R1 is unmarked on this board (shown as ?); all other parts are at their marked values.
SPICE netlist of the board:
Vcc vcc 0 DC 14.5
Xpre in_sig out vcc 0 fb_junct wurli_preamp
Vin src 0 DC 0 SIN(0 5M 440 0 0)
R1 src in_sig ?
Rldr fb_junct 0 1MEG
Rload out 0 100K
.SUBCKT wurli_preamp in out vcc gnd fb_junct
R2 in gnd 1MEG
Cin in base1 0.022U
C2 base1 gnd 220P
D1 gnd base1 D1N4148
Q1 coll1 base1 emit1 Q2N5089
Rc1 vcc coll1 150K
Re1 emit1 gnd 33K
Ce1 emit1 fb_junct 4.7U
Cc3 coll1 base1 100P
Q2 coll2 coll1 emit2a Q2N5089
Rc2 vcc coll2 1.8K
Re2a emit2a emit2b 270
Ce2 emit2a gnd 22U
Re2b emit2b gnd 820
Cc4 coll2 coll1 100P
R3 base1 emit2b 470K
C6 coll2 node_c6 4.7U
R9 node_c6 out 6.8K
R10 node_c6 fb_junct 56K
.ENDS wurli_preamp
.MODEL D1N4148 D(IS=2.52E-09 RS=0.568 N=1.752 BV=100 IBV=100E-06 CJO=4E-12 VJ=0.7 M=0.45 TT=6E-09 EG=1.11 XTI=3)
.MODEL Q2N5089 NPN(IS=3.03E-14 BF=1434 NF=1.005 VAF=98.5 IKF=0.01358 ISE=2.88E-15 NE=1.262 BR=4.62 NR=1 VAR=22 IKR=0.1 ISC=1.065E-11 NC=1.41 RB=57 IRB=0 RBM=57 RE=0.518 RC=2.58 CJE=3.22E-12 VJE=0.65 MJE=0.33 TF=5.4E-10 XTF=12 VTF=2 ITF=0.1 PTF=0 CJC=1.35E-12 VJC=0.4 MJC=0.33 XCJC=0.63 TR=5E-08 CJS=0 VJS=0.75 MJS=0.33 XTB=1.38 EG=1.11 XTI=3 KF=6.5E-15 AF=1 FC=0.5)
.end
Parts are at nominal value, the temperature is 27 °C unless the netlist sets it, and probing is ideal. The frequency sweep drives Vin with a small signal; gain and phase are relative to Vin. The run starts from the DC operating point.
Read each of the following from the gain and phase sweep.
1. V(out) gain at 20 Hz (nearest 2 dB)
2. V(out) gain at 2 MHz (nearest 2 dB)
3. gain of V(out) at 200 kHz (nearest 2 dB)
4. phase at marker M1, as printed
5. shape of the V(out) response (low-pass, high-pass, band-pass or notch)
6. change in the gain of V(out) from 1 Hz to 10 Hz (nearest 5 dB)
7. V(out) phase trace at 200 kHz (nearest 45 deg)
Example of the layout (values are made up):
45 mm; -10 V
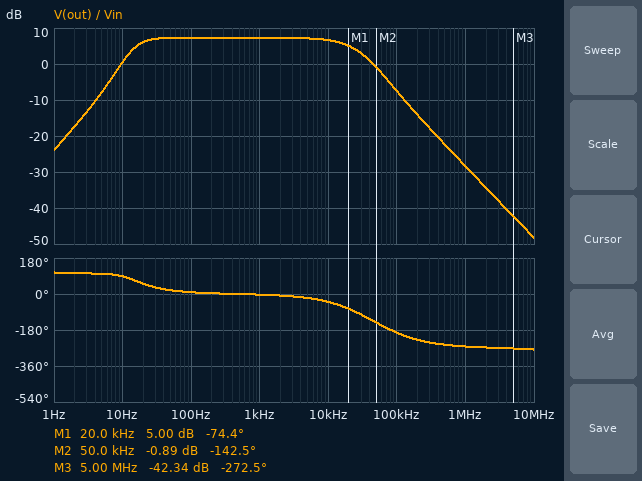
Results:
6 dB; -34 dB; -14 dB; -74.4 deg; band-pass; 25 dB; -225 deg
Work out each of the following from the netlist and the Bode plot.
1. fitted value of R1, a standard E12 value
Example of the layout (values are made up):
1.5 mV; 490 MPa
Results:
12 kΩ
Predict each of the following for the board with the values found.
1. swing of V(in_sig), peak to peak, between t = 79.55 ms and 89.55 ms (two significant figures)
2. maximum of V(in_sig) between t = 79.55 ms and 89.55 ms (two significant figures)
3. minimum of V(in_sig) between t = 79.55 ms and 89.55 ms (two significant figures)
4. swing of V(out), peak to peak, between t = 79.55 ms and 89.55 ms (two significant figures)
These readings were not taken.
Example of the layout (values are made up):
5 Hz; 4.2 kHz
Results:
9.6 mV; 4.8 mV; -4.8 mV; 23 mV
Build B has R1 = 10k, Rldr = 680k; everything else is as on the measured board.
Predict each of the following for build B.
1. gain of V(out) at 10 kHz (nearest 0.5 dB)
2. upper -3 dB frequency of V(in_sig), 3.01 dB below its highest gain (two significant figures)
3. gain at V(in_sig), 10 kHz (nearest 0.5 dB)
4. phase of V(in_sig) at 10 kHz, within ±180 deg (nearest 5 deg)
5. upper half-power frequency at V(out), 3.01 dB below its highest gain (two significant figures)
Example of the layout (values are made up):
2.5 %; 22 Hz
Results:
7.0 dB; 49 kHz; -0.5 dB; -10 deg; 25 kHz
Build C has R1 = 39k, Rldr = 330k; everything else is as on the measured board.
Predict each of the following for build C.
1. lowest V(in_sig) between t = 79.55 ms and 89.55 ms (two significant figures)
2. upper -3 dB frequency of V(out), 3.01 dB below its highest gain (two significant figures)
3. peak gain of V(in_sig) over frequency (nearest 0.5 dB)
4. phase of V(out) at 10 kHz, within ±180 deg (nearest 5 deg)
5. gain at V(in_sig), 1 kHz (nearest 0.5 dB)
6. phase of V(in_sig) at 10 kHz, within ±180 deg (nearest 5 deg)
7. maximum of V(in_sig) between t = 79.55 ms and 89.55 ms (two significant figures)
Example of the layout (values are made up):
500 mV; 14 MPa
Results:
-4.5 mV; 12 kHz; -0.5 dB; -60 deg; -1.0 dB; -35 deg; 4.5 mV
